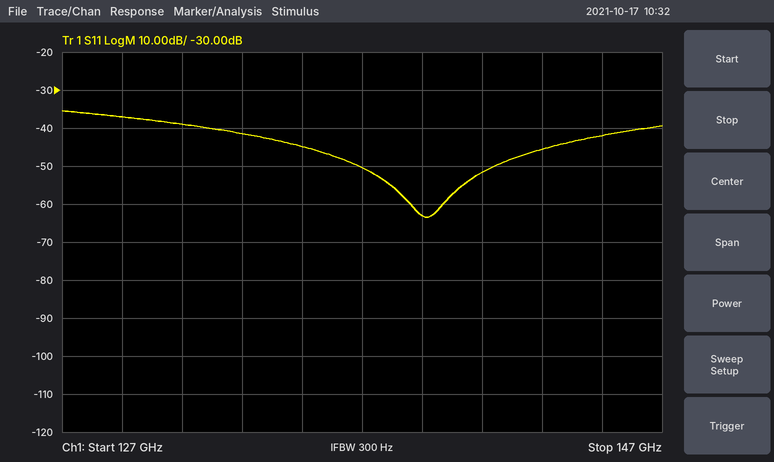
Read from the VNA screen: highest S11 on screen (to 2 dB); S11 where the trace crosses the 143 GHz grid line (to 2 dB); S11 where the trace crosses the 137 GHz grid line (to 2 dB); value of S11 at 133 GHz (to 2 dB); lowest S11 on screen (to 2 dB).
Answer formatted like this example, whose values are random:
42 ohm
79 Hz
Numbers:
-36 dB
-46 dB
-50 dB
-42 dB
-64 dB
